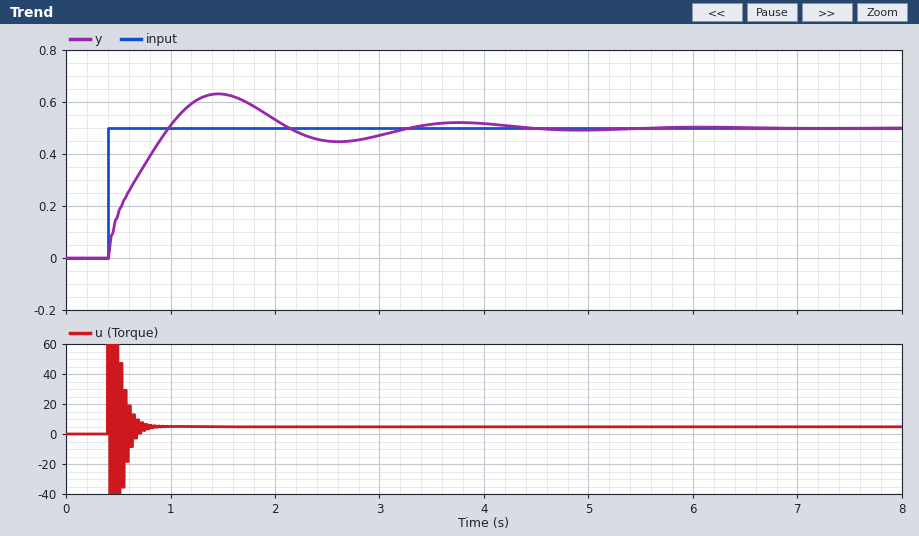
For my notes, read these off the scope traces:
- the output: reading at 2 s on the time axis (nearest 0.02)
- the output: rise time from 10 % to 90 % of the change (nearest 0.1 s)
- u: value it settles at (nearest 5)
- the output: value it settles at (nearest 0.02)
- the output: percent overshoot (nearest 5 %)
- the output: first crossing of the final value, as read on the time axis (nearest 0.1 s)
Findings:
0.54
0.5 s
5
0.50
25 %
1.0 s
